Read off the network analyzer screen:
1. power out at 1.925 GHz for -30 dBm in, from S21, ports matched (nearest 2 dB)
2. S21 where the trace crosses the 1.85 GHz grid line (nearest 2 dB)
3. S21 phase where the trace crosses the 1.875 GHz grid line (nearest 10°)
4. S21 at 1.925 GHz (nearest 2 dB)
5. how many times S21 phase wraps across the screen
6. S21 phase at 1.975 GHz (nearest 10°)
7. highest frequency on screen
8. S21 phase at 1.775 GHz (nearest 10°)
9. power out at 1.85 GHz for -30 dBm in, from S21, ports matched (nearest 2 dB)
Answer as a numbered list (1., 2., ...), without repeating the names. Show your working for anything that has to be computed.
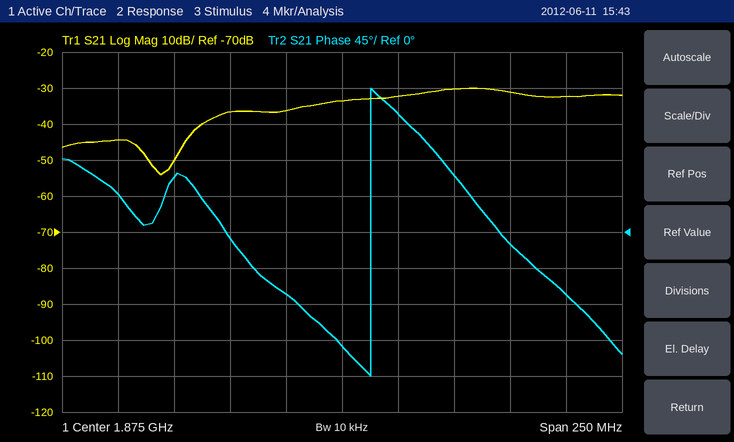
1. -30 dBm + (-30 dB) = -60 dBm
2. -36 dB
3. -140°
4. -30 dB
5. 1
6. -80°
7. 2 GHz
8. 50°
9. -30 dBm + (-36 dB) = -66 dBm
